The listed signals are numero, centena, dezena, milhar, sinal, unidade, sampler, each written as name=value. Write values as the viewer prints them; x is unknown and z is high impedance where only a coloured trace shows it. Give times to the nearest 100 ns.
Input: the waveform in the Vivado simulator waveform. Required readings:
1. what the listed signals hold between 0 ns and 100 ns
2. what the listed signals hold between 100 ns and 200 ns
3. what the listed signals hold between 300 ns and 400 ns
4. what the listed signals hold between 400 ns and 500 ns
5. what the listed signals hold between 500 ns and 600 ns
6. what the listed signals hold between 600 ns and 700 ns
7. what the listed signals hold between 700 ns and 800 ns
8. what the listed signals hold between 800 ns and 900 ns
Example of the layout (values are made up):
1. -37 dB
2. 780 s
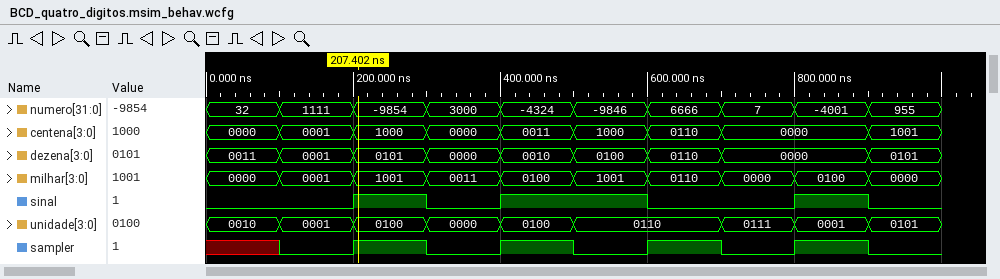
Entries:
1. numero=32, centena=0000, dezena=0011, milhar=0000, sinal=0, unidade=0010, sampler=x
2. numero=1111, centena=0001, dezena=0001, milhar=0001, sinal=0, unidade=0001, sampler=0
3. numero=3000, centena=0000, dezena=0000, milhar=0011, sinal=0, unidade=0000, sampler=0
4. numero=-4324, centena=0011, dezena=0010, milhar=0100, sinal=1, unidade=0100, sampler=1
5. numero=-9846, centena=1000, dezena=0100, milhar=1001, sinal=1, unidade=0110, sampler=0
6. numero=6666, centena=0110, dezena=0110, milhar=0110, sinal=0, unidade=0110, sampler=1
7. numero=7, centena=0000, dezena=0000, milhar=0000, sinal=0, unidade=0111, sampler=0
8. numero=-4001, centena=0000, dezena=0000, milhar=0100, sinal=1, unidade=0001, sampler=1
